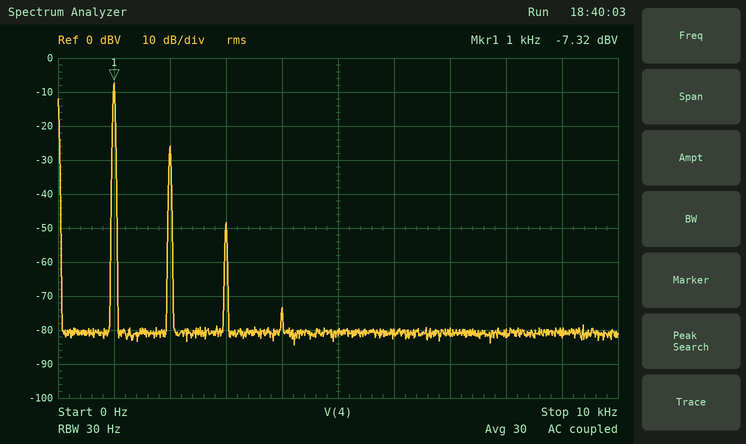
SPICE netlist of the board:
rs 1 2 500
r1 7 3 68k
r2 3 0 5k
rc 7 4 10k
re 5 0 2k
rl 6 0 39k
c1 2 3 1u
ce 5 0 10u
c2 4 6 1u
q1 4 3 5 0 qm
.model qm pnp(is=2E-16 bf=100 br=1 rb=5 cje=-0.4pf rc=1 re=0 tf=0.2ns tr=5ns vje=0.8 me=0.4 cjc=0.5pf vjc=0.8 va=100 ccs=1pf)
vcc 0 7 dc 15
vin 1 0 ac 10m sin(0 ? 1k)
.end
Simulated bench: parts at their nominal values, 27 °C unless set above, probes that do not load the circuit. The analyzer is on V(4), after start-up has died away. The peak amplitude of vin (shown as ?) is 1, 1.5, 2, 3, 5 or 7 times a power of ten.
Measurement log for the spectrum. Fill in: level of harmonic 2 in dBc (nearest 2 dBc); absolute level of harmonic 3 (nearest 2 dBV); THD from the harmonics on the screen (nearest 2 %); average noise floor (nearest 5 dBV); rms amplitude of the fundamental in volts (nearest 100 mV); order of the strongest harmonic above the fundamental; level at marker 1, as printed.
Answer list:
-18 dBc
-48 dBV
12 %
-80 dBV
400 mV
2
-7.32 dBV
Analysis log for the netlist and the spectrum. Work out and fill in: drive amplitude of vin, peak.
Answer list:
15 mV
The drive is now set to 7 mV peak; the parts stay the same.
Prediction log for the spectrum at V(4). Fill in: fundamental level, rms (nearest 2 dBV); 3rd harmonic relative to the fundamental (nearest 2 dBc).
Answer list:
-14 dBV
-54 dBc
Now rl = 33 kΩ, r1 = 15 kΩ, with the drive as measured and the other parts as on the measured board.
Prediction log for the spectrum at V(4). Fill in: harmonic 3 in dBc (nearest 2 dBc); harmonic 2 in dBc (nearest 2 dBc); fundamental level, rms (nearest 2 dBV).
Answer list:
-40 dBc
-20 dBc
-46 dBV
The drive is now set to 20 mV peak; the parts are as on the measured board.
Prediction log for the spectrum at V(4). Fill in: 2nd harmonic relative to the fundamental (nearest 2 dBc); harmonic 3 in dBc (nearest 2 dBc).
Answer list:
-16 dBc
-36 dBc
